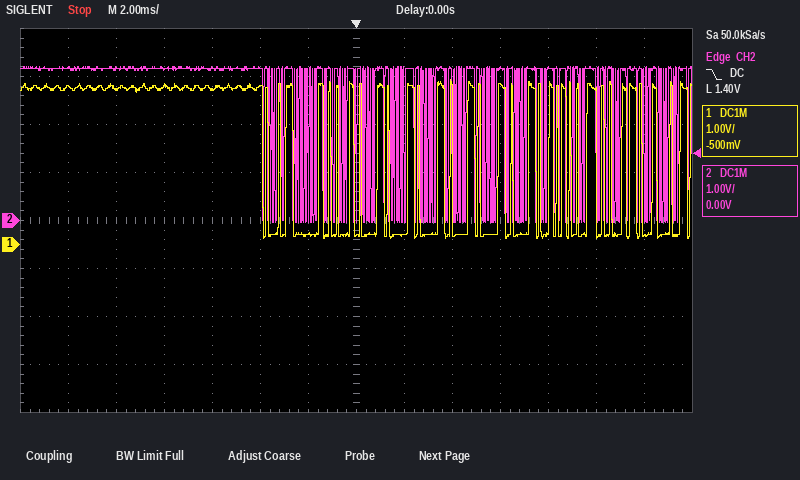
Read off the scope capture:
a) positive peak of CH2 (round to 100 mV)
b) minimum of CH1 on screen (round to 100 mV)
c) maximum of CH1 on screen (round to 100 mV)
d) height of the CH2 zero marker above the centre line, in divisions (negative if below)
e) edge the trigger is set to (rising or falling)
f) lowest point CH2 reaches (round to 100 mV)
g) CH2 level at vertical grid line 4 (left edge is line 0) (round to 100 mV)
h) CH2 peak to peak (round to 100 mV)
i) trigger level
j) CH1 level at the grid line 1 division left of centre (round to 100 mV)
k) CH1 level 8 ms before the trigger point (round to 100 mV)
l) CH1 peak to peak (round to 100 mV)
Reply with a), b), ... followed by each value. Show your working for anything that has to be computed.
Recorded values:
a) 3.2 V
b) 100 mV
c) 3.4 V
d) 0.0 div
e) falling
f) 0.0 V
g) 3.2 V
h) 3.2 V − (0.0 V) = 3.2 V
i) 1.40 V
j) 200 mV
k) 3.3 V
l) 3.4 V − (100 mV) = 3.3 V
